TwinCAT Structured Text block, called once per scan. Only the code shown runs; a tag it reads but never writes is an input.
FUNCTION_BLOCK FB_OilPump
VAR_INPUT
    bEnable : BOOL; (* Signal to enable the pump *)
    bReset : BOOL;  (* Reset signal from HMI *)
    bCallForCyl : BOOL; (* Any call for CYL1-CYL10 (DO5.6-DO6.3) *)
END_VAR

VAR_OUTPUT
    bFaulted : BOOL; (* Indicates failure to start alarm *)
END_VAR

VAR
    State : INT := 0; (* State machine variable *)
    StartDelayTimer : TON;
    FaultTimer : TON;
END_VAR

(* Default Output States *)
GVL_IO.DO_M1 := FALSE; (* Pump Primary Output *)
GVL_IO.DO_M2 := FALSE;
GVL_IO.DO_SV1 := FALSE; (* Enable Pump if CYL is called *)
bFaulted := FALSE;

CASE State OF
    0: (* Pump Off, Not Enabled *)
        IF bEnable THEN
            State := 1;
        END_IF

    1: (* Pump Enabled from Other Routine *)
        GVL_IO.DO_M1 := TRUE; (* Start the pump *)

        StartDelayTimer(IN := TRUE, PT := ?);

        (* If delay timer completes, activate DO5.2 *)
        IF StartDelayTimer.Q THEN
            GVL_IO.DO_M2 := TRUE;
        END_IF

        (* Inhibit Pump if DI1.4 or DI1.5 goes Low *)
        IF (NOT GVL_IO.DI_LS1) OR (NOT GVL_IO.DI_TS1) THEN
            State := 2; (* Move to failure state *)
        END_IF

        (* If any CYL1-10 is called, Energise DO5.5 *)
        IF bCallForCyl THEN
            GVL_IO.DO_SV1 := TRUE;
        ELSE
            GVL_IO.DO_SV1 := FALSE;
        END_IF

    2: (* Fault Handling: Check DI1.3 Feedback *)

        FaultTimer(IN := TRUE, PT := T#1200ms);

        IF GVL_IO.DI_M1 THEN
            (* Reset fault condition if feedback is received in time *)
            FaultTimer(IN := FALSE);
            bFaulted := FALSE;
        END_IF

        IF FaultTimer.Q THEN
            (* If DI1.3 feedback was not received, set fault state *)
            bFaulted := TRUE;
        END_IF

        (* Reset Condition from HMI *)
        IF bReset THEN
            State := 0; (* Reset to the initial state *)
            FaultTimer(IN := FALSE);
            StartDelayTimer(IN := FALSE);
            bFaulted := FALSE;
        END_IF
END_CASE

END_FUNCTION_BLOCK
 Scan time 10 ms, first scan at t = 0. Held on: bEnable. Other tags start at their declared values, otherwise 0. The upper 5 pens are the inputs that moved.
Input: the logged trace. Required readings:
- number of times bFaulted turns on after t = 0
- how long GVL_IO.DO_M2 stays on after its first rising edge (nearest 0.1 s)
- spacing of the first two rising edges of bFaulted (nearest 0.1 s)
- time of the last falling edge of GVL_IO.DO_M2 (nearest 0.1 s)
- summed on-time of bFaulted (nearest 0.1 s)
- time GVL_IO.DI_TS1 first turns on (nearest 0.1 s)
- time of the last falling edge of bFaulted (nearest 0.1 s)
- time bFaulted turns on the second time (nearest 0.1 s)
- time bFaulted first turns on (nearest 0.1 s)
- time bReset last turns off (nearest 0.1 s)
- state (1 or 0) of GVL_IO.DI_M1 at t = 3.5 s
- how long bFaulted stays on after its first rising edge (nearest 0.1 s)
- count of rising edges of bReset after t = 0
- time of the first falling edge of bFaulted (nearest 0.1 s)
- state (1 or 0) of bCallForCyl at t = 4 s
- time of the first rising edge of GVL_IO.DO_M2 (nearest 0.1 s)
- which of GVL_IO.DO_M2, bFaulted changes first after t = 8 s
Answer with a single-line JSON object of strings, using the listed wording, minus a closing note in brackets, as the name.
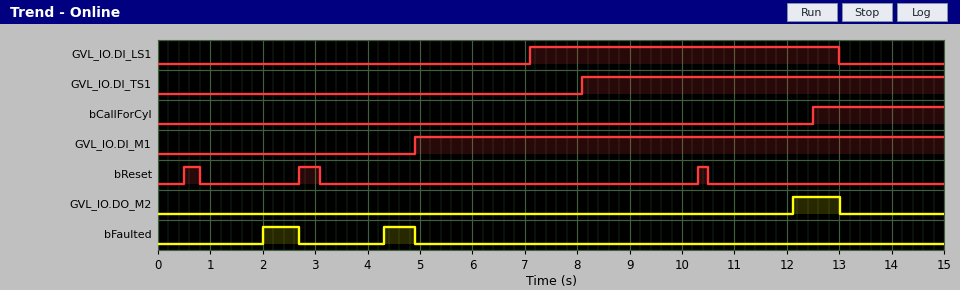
{"number of times bFaulted turns on after t = 0": "2", "how long GVL_IO.DO_M2 stays on after its first rising edge": "0.9 s", "spacing of the first two rising edges of bFaulted": "2.3 s", "time of the last falling edge of GVL_IO.DO_M2": "13.0 s", "summed on-time of bFaulted": "1.3 s", "time GVL_IO.DI_TS1 first turns on": "8.1 s", "time of the last falling edge of bFaulted": "4.9 s", "time bFaulted turns on the second time": "4.3 s", "time bFaulted first turns on": "2.0 s", "time bReset last turns off": "10.5 s", "state (1 or 0) of GVL_IO.DI_M1 at t = 3.5 s": "0", "how long bFaulted stays on after its first rising edge": "0.7 s", "count of rising edges of bReset after t = 0": "3", "time of the first falling edge of bFaulted": "2.7 s", "state (1 or 0) of bCallForCyl at t = 4 s": "0", "time of the first rising edge of GVL_IO.DO_M2": "12.1 s", "which of GVL_IO.DO_M2, bFaulted changes first after t = 8 s": "GVL_IO.DO_M2"}
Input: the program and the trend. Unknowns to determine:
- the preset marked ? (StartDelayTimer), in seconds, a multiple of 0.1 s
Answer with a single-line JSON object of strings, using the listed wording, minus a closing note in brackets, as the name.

{"the preset marked ? (StartDelayTimer), in seconds, a multiple of 0.1 s": "1.8 s"}
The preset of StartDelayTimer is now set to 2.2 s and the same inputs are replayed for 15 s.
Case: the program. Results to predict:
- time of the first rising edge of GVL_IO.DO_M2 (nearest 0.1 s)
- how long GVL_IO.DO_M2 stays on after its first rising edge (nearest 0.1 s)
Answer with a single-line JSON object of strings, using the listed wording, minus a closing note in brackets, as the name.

{"time of the first rising edge of GVL_IO.DO_M2": "12.5 s", "how long GVL_IO.DO_M2 stays on after its first rising edge": "0.5 s"}
